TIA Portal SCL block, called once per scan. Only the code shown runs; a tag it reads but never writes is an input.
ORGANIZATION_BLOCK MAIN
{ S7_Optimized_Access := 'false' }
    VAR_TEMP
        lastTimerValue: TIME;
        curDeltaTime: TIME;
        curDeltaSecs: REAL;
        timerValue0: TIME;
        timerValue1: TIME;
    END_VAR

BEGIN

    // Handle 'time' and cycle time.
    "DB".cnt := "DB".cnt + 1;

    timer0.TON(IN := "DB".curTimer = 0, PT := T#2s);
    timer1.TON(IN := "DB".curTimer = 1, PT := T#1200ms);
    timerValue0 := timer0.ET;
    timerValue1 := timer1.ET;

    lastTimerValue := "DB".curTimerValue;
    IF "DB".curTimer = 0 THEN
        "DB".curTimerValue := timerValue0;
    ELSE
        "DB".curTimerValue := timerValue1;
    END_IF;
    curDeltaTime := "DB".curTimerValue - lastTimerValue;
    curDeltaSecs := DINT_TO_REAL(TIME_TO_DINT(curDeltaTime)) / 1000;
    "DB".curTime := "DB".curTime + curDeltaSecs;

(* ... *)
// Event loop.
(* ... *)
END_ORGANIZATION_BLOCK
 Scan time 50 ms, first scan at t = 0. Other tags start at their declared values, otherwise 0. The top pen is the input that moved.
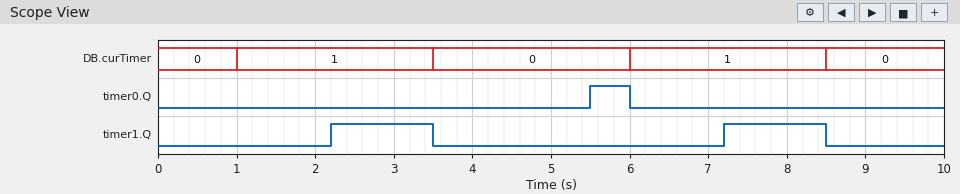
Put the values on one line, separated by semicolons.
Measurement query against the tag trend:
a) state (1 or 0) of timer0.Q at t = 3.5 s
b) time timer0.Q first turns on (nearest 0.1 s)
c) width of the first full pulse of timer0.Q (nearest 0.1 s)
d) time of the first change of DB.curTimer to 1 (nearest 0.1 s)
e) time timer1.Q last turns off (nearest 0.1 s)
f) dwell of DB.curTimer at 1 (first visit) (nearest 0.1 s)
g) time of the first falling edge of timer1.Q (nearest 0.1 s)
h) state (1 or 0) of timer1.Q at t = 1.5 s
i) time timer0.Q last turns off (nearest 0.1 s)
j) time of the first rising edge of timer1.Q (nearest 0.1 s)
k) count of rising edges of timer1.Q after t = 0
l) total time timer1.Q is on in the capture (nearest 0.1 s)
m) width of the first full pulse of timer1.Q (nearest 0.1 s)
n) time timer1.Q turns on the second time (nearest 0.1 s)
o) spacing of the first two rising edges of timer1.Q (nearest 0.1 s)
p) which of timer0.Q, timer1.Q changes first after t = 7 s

0; 5.5 s; 0.5 s; 1.0 s; 8.5 s; 2.5 s; 3.5 s; 0; 6.0 s; 2.2 s; 2; 2.6 s; 1.3 s; 7.2 s; 5.0 s; timer1.Q
